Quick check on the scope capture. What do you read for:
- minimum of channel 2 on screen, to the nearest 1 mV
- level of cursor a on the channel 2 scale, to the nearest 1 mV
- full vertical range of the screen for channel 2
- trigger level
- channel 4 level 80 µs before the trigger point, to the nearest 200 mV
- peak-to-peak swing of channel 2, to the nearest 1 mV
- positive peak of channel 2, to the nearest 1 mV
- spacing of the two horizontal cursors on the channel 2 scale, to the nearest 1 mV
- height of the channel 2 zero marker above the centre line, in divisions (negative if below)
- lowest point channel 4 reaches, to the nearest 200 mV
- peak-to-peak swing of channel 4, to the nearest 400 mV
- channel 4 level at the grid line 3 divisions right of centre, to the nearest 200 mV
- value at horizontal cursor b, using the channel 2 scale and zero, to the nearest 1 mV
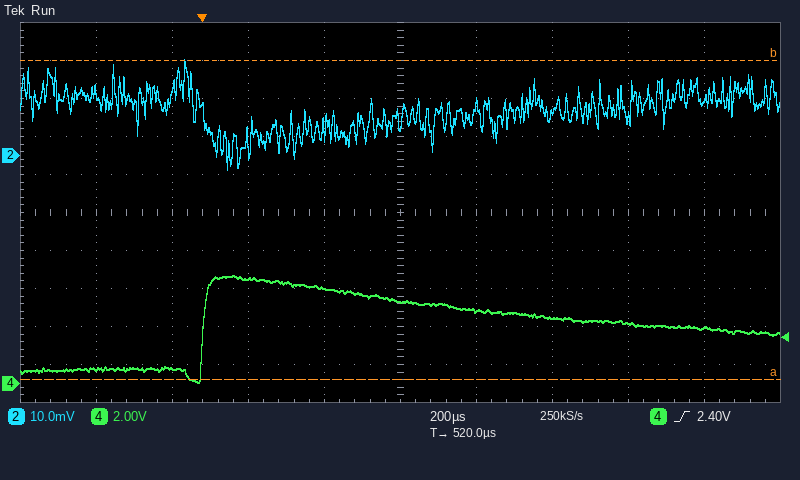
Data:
-4 mV
-59 mV
100 mV
2.40 V
800 mV
29 mV
25 mV
84 mV
+1.5 div
0.0 V
5.6 V
3.2 V
25 mV
